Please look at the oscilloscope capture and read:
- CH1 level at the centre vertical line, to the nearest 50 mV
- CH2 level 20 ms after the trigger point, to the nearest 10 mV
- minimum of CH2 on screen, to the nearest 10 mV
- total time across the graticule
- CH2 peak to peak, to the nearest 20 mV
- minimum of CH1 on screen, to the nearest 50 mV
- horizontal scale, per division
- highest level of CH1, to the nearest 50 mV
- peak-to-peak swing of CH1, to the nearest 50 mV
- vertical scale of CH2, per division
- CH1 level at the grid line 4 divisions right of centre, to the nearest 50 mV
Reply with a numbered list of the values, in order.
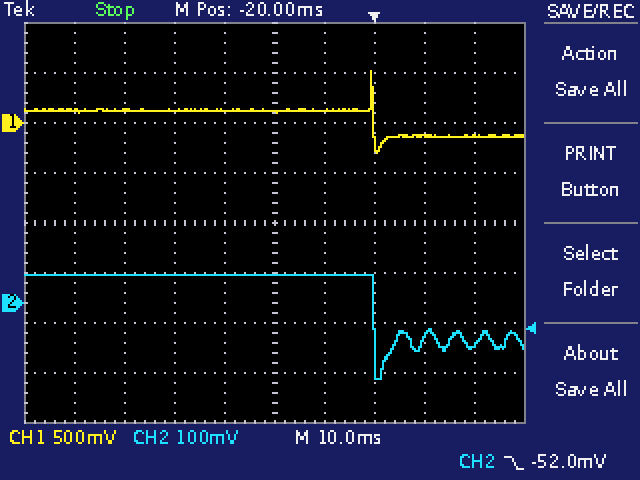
1. 100 mV
2. -80 mV
3. -150 mV
4. 100 ms
5. 200 mV
6. -300 mV
7. 10 ms
8. 500 mV
9. 800 mV
10. 100 mV
11. -150 mV
